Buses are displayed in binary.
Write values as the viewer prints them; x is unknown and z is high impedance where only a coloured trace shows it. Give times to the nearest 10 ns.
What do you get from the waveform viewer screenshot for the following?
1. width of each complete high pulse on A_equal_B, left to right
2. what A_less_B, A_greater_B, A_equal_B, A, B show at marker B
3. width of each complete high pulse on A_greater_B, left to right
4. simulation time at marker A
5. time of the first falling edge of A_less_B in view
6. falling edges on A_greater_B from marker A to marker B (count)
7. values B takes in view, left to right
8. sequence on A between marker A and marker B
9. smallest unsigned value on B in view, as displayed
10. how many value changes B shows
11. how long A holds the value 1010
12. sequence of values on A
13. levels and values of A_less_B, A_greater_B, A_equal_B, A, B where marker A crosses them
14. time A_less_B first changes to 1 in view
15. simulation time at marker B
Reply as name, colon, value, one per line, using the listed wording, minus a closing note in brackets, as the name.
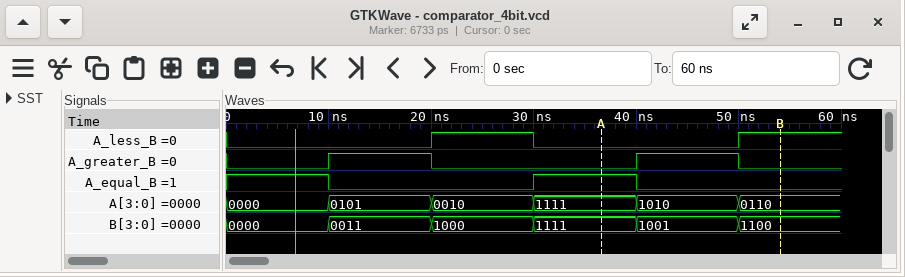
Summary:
width of each complete high pulse on A_equal_B, left to right: 10 ns
what A_less_B, A_greater_B, A_equal_B, A, B show at marker B: A_less_B=1, A_greater_B=0, A_equal_B=0, A=0110, B=1100
width of each complete high pulse on A_greater_B, left to right: 10 ns, 10 ns
simulation time at marker A: 40 ns
time of the first falling edge of A_less_B in view: 30 ns
falling edges on A_greater_B from marker A to marker B: 1
values B takes in view, left to right: 0000, 0011, 1000, 1111, 1001, 1100
sequence on A between marker A and marker B: 1111, 1010, 0110
smallest unsigned value on B in view, as displayed: 0000
how many value changes B shows: 5
how long A holds the value 1010: 10 ns
sequence of values on A: 0000, 0101, 0010, 1111, 1010, 0110
levels and values of A_less_B, A_greater_B, A_equal_B, A, B where marker A crosses them: A_less_B=0, A_greater_B=0, A_equal_B=1, A=1111, B=1111
time A_less_B first changes to 1 in view: 20 ns
simulation time at marker B: 50 ns
